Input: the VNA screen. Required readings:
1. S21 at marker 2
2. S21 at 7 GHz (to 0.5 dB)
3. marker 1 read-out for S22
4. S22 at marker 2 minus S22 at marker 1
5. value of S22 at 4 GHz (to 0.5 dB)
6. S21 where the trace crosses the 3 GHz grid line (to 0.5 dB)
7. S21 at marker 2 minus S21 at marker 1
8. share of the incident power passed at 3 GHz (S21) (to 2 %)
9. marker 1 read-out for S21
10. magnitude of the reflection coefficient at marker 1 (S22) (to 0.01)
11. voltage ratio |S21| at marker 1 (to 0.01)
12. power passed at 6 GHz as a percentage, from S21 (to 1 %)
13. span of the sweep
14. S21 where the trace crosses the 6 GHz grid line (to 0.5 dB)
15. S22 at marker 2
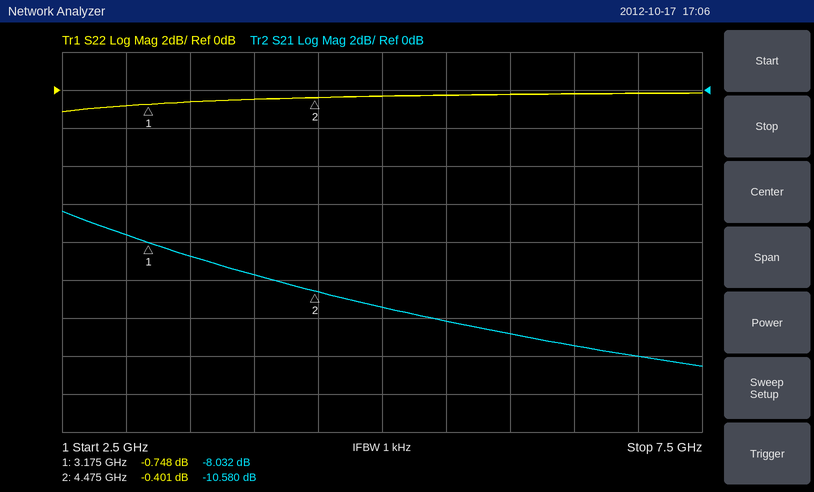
-10.580 dB
-14.0 dB
-0.748 dB
0.347 dB
-0.5 dB
-7.5 dB
-2.548 dB
18 %
-8.032 dB
0.92
0.40
5 %
5 GHz
-13.0 dB
-0.401 dB
